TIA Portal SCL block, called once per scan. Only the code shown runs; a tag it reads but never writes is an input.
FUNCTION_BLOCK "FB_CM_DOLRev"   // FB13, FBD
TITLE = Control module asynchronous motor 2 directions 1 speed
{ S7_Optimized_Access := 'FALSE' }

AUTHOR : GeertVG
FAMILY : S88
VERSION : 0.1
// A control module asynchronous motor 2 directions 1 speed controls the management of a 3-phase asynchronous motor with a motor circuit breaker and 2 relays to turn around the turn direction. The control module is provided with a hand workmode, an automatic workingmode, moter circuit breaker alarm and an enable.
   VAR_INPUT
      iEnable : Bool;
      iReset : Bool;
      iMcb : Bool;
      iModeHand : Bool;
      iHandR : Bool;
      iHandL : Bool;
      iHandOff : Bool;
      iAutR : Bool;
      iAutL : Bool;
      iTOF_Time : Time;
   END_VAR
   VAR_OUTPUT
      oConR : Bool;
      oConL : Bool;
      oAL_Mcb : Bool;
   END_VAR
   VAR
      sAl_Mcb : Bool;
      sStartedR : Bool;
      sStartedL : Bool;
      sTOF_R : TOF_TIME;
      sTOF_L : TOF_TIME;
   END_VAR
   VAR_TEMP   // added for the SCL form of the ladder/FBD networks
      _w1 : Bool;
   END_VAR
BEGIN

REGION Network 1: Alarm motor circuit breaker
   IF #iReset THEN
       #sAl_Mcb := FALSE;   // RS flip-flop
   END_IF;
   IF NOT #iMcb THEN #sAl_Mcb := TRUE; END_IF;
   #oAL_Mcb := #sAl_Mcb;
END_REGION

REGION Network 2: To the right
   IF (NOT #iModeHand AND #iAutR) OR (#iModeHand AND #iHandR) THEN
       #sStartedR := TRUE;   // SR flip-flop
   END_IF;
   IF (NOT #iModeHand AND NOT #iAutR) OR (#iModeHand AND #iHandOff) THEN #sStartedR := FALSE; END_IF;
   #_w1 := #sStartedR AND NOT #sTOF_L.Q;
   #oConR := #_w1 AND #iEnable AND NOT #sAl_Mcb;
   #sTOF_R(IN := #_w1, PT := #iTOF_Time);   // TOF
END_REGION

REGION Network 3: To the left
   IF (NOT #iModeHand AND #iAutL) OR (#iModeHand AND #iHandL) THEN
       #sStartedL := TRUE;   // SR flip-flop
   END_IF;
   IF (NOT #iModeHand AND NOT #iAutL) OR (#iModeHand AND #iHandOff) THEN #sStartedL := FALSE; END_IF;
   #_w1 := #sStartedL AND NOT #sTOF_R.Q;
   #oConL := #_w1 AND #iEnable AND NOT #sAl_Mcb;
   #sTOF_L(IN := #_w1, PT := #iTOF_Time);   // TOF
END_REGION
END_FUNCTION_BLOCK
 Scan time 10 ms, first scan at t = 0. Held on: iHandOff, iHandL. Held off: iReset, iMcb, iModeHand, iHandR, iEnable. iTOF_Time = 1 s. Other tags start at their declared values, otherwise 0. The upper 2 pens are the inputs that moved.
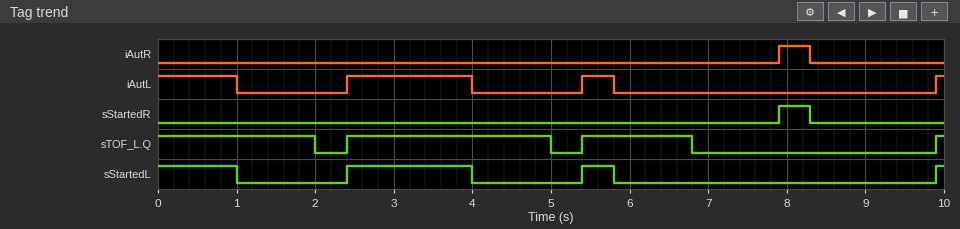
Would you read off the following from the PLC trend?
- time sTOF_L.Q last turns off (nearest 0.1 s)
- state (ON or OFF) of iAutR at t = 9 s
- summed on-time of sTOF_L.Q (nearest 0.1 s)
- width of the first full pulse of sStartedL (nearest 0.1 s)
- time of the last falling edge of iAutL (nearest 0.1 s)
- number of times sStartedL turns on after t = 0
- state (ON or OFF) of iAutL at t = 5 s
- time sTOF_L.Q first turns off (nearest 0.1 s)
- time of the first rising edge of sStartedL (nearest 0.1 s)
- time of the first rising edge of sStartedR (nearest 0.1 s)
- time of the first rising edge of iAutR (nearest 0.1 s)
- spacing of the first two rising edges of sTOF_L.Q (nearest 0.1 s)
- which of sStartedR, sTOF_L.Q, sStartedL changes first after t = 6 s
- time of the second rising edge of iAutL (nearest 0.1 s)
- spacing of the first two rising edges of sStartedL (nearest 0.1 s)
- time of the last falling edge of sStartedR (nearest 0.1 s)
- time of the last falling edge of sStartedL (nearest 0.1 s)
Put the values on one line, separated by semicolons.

6.8 s; OFF; 6.1 s; 1.6 s; 5.8 s; 3; OFF; 2.0 s; 2.4 s; 7.9 s; 7.9 s; 3.0 s; sTOF_L.Q; 5.4 s; 3.0 s; 8.3 s; 5.8 s
